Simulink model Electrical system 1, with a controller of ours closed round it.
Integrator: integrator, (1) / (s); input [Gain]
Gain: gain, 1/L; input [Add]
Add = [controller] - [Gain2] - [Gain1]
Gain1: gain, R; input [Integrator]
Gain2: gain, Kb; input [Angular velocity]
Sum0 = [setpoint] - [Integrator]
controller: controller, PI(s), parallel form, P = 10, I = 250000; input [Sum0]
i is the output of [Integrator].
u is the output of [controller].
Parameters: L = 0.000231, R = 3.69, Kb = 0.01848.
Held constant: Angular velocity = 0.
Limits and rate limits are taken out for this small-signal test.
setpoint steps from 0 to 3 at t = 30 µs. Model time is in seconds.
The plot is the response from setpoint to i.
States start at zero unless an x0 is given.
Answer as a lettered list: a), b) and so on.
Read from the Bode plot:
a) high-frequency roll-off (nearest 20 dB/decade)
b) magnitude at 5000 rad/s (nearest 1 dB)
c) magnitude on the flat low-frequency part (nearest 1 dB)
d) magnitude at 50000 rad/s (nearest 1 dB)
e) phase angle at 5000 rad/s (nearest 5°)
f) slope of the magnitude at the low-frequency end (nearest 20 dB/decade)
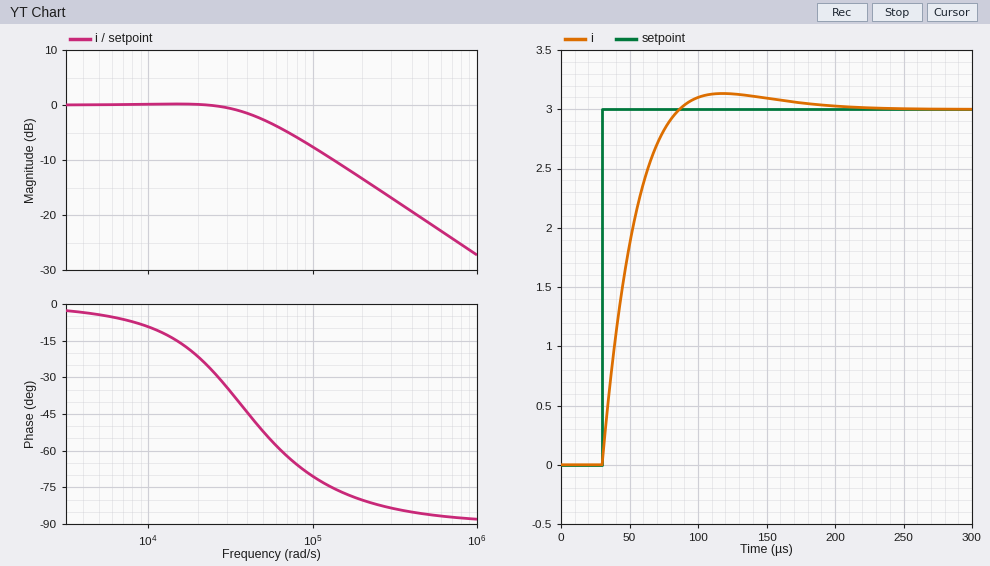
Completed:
a) -20 dB/decade
b) 0 dB
c) 0 dB
d) -3 dB
e) -5°
f) 0 dB/decade
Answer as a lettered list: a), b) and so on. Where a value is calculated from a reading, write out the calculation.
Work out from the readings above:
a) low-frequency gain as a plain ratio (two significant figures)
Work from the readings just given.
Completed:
a) 10^(0 / 20) = 1.0
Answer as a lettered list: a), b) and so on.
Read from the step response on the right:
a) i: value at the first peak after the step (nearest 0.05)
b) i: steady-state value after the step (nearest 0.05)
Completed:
a) 3.15
b) 3.00
